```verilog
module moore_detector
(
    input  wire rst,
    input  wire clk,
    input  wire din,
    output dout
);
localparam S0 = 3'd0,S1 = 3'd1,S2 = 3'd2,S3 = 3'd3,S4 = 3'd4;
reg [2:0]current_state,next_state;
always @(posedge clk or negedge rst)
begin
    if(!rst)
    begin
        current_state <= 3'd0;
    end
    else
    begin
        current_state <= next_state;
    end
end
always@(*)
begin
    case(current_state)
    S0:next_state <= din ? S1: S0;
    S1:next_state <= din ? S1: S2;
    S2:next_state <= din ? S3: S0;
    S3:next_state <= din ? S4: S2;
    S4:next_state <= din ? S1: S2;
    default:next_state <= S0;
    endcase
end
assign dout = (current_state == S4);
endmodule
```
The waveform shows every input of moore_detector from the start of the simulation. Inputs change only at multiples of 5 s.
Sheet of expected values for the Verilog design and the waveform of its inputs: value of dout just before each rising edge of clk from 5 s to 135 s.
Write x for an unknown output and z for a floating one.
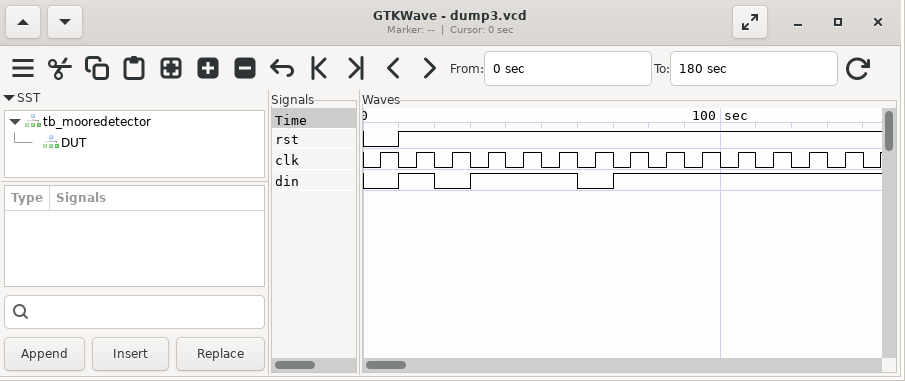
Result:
0 0 0 0 0 1 0 0 0 1 0 0 0 0
